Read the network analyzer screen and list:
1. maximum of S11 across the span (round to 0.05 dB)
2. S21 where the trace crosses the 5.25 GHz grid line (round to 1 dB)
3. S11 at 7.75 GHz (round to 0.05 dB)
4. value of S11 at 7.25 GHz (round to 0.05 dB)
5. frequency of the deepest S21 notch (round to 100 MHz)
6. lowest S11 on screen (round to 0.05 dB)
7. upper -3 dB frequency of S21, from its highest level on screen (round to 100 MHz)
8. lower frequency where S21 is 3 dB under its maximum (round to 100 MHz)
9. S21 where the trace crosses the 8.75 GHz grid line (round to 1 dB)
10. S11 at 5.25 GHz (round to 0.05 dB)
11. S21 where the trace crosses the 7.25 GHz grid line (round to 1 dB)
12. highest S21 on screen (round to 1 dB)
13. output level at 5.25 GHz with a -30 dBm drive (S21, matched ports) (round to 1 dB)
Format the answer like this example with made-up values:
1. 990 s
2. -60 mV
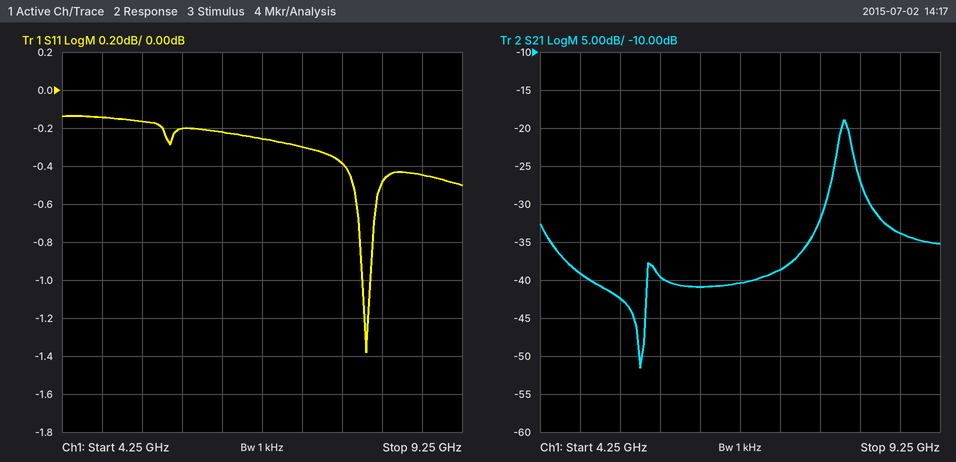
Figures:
1. -0.15 dB
2. -42 dB
3. -0.40 dB
4. -0.30 dB
5. 5.5 GHz
6. -1.40 dB
7. 8.1 GHz
8. 8.0 GHz
9. -34 dB
10. -0.15 dB
11. -39 dB
12. -19 dB
13. -72 dBm
